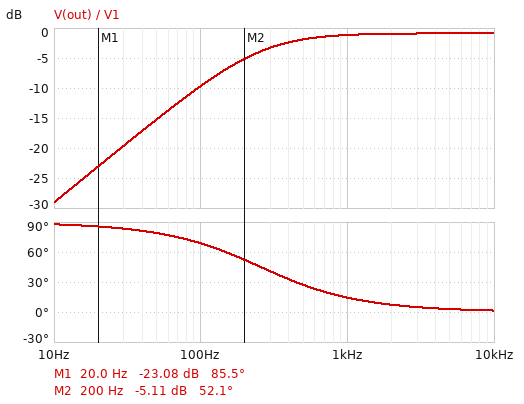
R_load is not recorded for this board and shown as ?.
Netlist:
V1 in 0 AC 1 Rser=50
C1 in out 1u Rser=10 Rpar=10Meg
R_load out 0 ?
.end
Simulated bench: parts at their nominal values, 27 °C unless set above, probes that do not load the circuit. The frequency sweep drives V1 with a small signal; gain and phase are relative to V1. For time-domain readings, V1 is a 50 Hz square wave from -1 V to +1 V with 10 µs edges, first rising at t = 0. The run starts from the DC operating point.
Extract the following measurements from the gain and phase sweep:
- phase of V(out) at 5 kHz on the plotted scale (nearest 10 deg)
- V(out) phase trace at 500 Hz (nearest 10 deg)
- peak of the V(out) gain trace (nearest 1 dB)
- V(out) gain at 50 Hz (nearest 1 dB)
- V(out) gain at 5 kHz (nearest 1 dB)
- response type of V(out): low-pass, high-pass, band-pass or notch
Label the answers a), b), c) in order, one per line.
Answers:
a) 0 deg
b) 30 deg
c) -1 dB
d) -15 dB
e) -1 dB
f) high-pass
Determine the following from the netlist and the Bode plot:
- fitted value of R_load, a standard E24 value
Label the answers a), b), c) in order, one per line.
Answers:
a) 560 Ω
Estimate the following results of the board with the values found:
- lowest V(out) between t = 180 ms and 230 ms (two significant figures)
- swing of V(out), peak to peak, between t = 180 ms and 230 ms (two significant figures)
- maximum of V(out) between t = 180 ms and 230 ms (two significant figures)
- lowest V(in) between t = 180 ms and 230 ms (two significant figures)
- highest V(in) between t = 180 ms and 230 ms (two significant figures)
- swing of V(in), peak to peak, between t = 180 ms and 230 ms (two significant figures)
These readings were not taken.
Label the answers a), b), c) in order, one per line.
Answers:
a) -1.8 V
b) 3.6 V
c) 1.8 V
d) -1.0 V
e) 1.0 V
f) 2.0 V
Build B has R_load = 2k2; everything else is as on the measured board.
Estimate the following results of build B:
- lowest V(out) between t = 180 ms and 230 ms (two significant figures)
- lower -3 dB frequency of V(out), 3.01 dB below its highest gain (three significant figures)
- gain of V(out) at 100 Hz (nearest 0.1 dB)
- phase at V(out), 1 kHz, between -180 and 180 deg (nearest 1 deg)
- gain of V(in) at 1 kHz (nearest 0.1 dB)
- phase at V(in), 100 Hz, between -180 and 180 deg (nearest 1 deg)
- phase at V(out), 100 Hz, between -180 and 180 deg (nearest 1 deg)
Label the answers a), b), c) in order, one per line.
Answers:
a) -1.9 V
b) 70.4 Hz
c) -2.0 dB
d) 4 deg
e) -0.2 dB
f) -1 deg
g) 35 deg
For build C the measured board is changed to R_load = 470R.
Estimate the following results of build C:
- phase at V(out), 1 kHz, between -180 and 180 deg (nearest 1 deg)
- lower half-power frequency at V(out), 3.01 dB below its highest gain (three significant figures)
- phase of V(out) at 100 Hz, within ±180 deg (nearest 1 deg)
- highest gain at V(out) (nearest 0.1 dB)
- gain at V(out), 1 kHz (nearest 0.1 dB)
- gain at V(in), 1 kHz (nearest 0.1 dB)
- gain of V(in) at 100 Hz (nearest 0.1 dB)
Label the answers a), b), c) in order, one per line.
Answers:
a) 17 deg
b) 300 Hz
c) 72 deg
d) -1.0 dB
e) -1.4 dB
f) -0.8 dB
g) -0.1 dB
